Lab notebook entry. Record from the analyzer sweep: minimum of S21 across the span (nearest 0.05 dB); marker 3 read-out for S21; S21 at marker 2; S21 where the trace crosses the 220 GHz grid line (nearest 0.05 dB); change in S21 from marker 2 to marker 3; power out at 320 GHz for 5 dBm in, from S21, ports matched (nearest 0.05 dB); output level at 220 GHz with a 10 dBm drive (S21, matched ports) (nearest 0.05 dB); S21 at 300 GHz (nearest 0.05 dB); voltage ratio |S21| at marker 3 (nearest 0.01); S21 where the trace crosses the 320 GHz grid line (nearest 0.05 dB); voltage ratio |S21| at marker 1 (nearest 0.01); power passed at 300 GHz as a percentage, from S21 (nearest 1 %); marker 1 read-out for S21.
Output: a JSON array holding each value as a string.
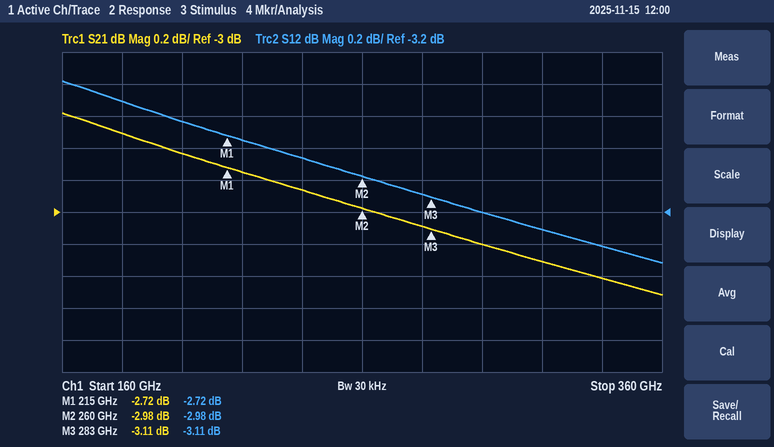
["-3.50 dB", "-3.11 dB", "-2.98 dB", "-2.75 dB", "-0.13 dB", "1.70 dBm", "7.25 dBm", "-3.20 dB", "0.70", "-3.30 dB", "0.73", "48 %", "-2.72 dB"]
